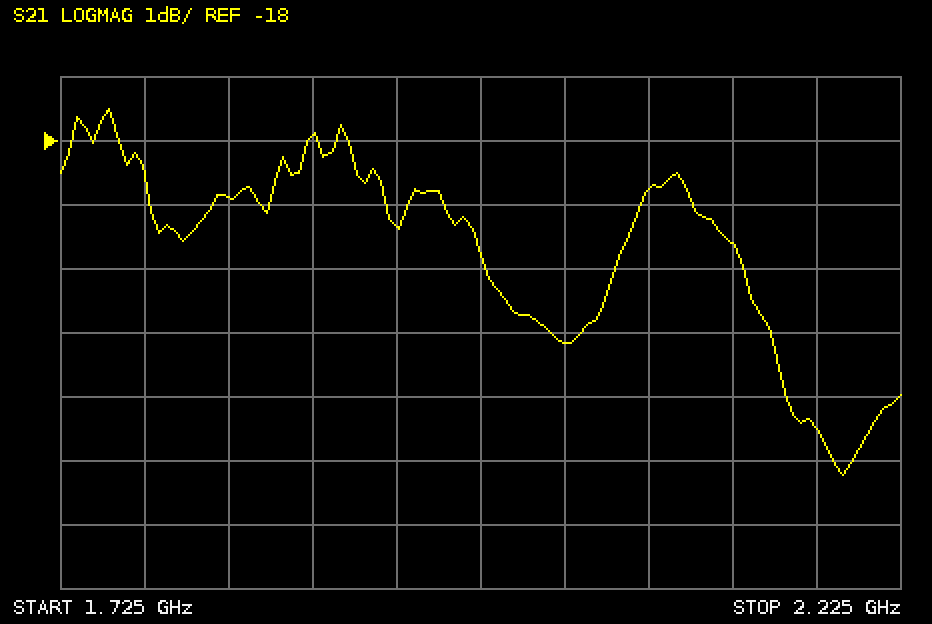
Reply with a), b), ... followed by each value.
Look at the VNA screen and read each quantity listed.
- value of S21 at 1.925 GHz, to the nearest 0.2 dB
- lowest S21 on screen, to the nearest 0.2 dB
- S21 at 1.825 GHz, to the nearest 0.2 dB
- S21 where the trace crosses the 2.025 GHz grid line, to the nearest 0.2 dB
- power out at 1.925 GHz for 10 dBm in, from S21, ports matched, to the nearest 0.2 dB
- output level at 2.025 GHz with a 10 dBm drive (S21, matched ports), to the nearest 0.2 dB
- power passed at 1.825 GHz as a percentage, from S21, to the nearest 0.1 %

a) -19.4 dB
b) -23.2 dB
c) -18.8 dB
d) -21.2 dB
e) -9.4 dBm
f) -11.2 dBm
g) 1.3 %
